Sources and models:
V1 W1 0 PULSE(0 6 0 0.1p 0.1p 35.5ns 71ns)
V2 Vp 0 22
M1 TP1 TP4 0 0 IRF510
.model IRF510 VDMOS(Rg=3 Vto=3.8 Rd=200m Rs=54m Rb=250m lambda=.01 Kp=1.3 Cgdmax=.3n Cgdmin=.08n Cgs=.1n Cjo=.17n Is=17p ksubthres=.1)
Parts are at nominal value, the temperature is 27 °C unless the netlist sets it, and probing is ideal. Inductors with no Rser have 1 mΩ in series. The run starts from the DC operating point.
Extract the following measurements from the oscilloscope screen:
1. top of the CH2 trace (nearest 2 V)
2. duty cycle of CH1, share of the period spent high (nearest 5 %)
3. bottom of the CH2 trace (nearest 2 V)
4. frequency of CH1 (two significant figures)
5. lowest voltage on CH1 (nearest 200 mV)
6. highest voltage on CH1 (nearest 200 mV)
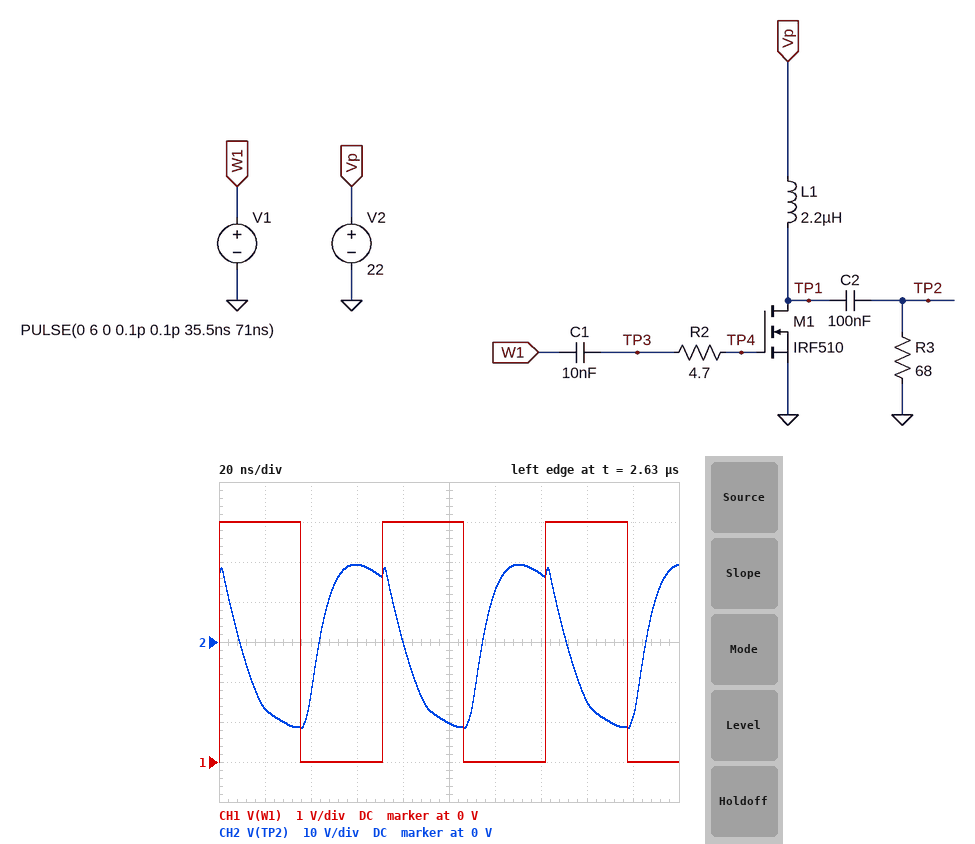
20 V
50 %
-22 V
14 MHz
0 V
6.0 V
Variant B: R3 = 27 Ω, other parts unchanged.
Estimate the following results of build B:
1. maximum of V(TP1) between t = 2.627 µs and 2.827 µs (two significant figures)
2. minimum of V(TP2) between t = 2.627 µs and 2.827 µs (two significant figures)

36 V
-19 V
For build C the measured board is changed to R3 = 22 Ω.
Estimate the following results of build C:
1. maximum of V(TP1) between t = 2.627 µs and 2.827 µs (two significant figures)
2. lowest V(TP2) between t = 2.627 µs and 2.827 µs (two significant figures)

35 V
-18 V
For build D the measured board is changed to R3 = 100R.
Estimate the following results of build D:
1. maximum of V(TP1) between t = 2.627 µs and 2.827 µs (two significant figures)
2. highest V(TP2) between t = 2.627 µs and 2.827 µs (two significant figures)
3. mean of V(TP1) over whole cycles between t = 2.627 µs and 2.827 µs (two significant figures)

44 V
22 V
22 V
